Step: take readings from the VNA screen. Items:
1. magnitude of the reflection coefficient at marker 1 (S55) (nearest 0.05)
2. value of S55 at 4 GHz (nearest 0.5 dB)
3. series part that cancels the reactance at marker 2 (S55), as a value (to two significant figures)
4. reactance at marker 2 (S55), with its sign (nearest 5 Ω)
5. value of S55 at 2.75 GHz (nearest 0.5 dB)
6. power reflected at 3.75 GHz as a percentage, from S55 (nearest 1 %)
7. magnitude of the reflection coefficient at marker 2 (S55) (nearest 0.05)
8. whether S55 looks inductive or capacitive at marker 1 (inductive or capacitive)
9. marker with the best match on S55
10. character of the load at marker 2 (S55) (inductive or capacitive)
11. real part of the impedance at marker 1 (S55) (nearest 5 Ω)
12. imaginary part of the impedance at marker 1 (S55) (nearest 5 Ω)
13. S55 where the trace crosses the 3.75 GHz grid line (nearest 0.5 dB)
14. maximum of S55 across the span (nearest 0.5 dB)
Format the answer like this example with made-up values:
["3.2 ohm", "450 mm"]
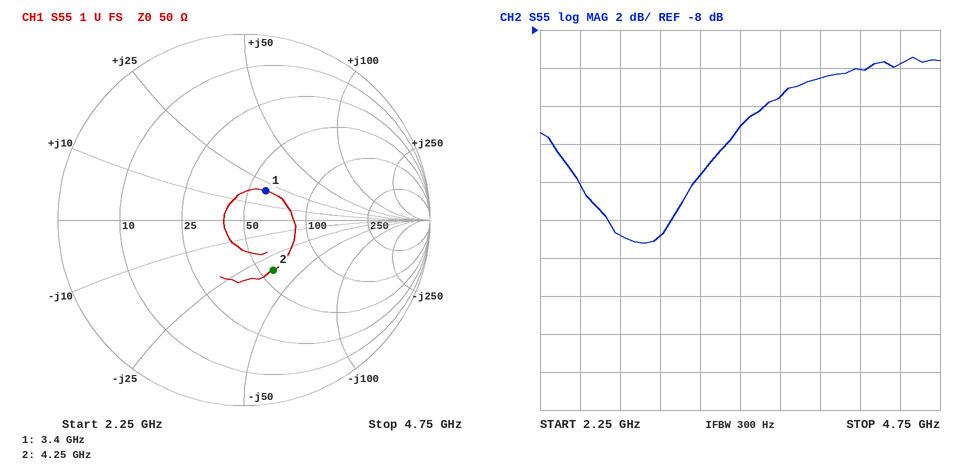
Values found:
["0.20", "-10.5 dB", "1.3 nH", "-35 Ω", "-19.0 dB", "7 %", "0.30", "inductive", "marker 1", "capacitive", "60 Ω", "+20 Ω", "-11.5 dB", "-9.5 dB"]
